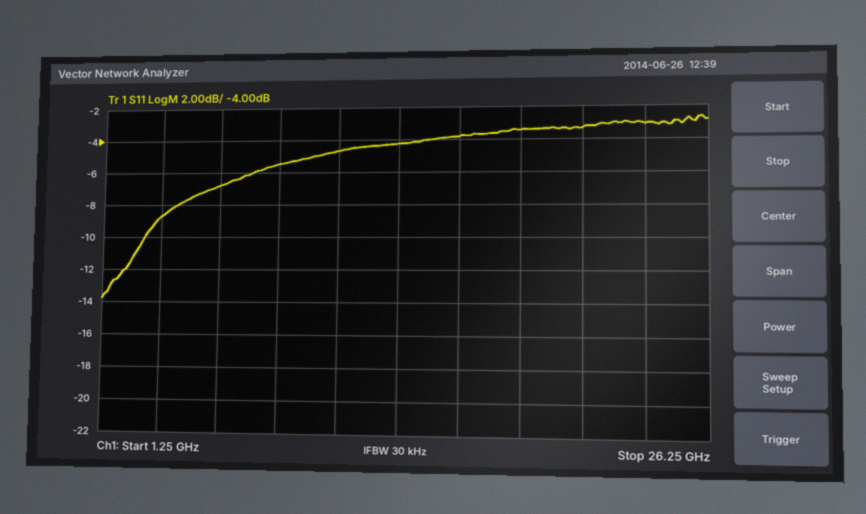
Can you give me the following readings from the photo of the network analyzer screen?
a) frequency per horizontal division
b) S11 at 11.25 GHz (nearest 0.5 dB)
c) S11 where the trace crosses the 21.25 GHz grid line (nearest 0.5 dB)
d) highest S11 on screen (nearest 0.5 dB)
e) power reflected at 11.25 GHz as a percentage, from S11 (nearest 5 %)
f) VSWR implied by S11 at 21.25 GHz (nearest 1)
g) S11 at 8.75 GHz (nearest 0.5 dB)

2.5 GHz
-4.5 dB
-3.5 dB
-2.5 dB
35 %
5
-5.5 dB
